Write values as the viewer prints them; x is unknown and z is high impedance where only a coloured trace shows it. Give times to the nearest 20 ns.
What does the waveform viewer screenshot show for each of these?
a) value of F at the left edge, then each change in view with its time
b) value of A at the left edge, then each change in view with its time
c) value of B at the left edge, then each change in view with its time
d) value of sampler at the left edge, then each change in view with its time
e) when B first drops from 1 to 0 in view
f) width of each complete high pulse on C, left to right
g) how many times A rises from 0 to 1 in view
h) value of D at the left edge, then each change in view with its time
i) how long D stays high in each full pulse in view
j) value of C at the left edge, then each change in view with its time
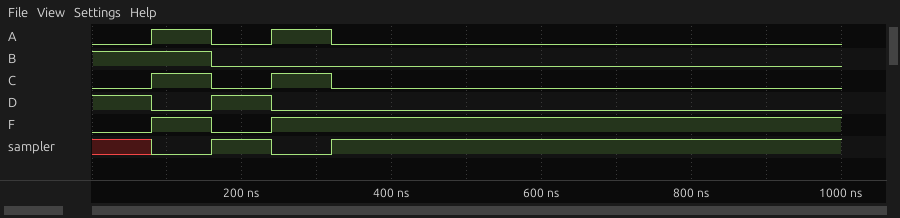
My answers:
0, 1 at 80 ns, 0 at 160 ns, 1 at 240 ns
0, 1 at 80 ns, 0 at 160 ns, 1 at 240 ns, 0 at 320 ns
1, 0 at 160 ns
x, 0 at 80 ns, 1 at 160 ns, 0 at 240 ns, 1 at 320 ns
160 ns
80 ns, 80 ns
2
1, 0 at 80 ns, 1 at 160 ns, 0 at 240 ns
80 ns
0, 1 at 80 ns, 0 at 160 ns, 1 at 240 ns, 0 at 320 ns
